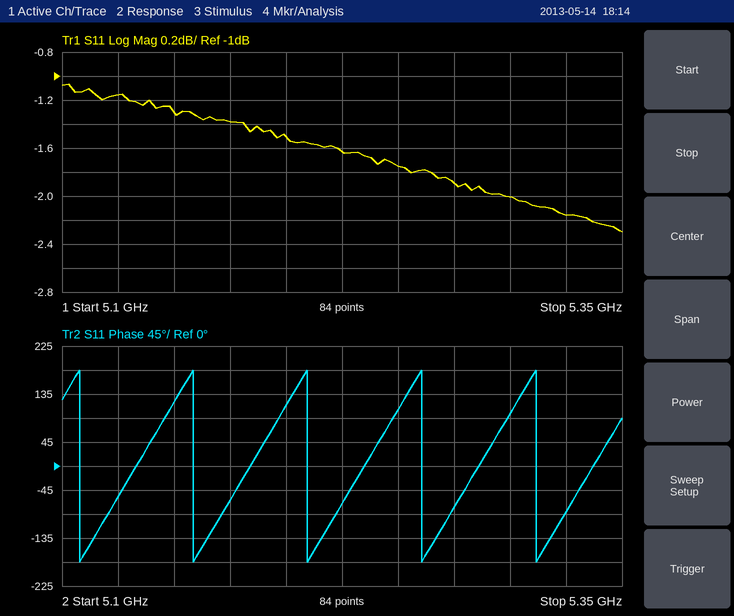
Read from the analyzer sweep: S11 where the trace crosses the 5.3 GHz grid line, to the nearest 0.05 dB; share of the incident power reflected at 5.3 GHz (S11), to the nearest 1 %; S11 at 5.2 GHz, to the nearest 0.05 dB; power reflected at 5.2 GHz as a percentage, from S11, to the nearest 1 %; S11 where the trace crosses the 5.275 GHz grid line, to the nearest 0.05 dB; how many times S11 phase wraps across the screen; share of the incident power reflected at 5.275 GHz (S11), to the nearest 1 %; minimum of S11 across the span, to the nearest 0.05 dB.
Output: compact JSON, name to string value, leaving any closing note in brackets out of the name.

{"S11 where the trace crosses the 5.3 GHz grid line, to the nearest 0.05 dB": "-2.00 dB", "share of the incident power reflected at 5.3 GHz (S11), to the nearest 1 %": "63 %", "S11 at 5.2 GHz, to the nearest 0.05 dB": "-1.50 dB", "power reflected at 5.2 GHz as a percentage, from S11, to the nearest 1 %": "71 %", "S11 where the trace crosses the 5.275 GHz grid line, to the nearest 0.05 dB": "-1.90 dB", "how many times S11 phase wraps across the screen": "5", "share of the incident power reflected at 5.275 GHz (S11), to the nearest 1 %": "65 %", "minimum of S11 across the span, to the nearest 0.05 dB": "-2.30 dB"}
